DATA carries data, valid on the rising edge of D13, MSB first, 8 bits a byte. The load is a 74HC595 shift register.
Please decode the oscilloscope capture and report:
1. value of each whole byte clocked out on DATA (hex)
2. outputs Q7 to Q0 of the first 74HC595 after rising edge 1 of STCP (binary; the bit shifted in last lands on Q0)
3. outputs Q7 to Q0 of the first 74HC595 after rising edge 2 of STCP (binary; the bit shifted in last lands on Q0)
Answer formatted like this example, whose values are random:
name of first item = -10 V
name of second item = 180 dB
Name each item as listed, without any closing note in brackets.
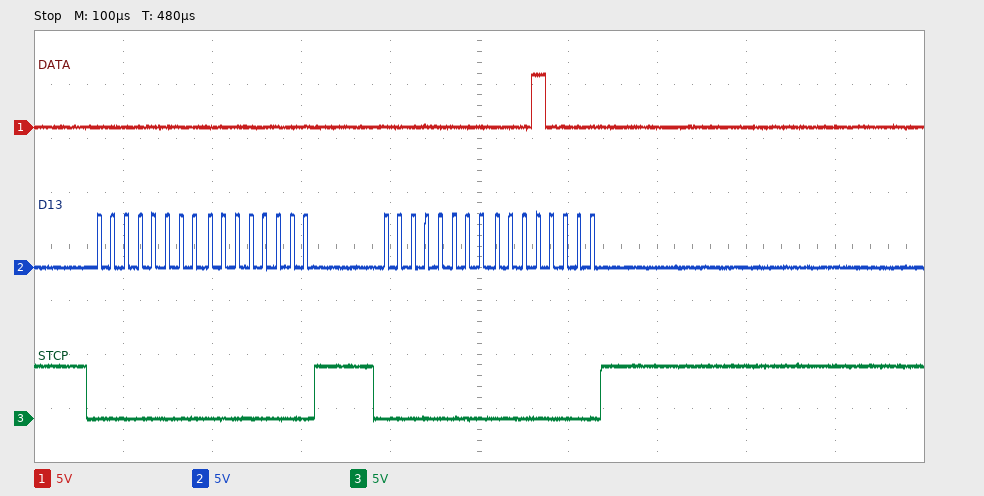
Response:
value of each whole byte clocked out on DATA = 0x00 0x00 0x00 0x10
outputs Q7 to Q0 of the first 74HC595 after rising edge 1 of STCP = 00000000
outputs Q7 to Q0 of the first 74HC595 after rising edge 2 of STCP = 00010000
